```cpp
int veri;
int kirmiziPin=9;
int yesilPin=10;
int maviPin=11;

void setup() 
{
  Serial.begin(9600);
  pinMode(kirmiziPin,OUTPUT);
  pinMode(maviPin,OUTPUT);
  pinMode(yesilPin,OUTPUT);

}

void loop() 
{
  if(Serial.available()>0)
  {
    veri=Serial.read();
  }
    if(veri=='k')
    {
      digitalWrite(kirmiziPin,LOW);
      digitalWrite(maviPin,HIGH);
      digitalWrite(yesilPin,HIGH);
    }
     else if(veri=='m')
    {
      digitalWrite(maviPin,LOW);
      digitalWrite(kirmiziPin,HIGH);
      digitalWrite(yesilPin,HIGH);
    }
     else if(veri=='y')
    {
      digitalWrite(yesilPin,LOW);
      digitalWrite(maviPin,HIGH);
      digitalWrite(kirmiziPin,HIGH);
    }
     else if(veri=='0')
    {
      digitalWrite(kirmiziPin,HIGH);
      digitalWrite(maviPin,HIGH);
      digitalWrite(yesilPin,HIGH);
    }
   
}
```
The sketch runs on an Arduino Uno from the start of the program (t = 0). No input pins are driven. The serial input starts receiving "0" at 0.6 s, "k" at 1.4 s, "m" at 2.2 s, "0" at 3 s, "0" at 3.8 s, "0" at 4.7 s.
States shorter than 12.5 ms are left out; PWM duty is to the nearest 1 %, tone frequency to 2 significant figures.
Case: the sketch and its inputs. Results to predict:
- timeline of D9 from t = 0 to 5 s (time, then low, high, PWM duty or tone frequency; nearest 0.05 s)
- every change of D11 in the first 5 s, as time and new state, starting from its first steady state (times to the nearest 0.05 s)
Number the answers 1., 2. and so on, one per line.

1. 0 s low; 0.6 s high; 1.4 s low; 2.2 s high
2. 0 s low; 0.6 s high; 2.2 s low; 3 s high
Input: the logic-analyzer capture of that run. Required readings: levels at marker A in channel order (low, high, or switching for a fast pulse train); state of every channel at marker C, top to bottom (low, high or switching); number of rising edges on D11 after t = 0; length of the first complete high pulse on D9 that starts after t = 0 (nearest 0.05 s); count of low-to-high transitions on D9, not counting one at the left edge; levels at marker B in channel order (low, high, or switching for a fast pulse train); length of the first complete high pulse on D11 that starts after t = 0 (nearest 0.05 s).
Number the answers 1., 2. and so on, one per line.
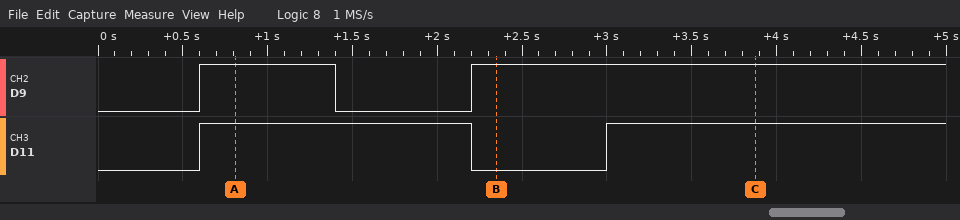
1. D9 high, D11 high
2. D9 high, D11 high
3. 2
4. 0.80 s
5. 2
6. D9 high, D11 low
7. 1.60 s
